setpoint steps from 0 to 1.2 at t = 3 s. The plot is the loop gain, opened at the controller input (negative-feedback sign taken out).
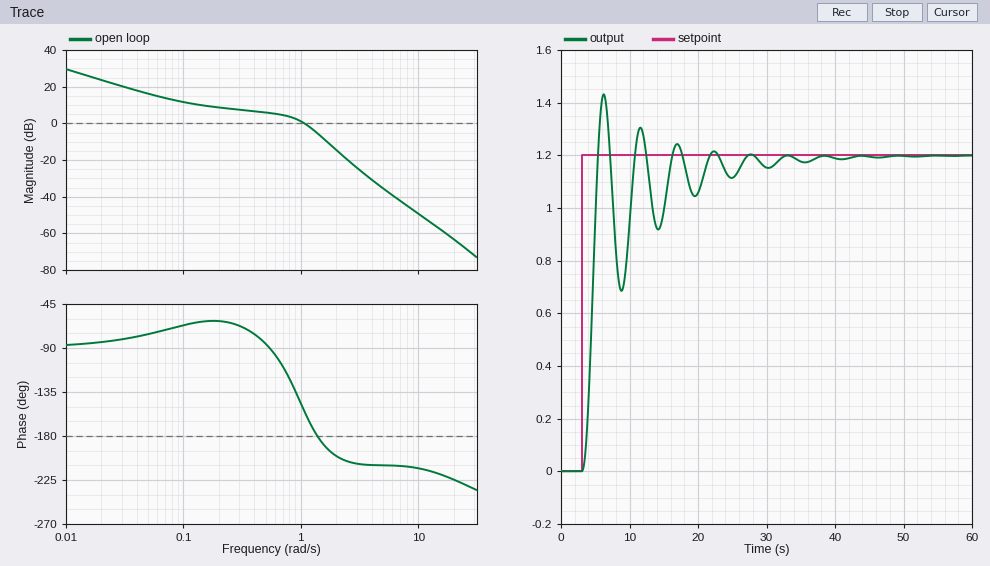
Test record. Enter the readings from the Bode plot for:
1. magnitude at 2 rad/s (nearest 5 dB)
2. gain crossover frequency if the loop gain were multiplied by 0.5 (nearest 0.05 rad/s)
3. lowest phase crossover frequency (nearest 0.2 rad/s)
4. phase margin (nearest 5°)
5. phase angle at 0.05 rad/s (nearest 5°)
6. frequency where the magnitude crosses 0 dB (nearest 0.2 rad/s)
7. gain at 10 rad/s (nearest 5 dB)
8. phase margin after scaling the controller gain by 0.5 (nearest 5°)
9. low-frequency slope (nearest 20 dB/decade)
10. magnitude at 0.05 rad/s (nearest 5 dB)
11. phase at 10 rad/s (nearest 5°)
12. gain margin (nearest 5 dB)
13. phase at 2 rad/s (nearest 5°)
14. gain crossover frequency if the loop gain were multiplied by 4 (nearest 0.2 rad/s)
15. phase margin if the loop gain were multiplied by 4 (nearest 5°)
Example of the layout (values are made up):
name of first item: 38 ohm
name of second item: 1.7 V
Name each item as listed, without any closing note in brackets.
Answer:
magnitude at 2 rad/s: -15 dB
gain crossover frequency if the loop gain were multiplied by 0.5: 0.50 rad/s
lowest phase crossover frequency: 1.4 rad/s
phase margin: 25°
phase angle at 0.05 rad/s: -75°
frequency where the magnitude crosses 0 dB: 1.0 rad/s
gain at 10 rad/s: -50 dB
phase margin after scaling the controller gain by 0.5: 95°
low-frequency slope: -20 dB/decade
magnitude at 0.05 rad/s: 15 dB
phase at 10 rad/s: -215°
gain margin: 5 dB
phase at 2 rad/s: -200°
gain crossover frequency if the loop gain were multiplied by 4: 1.8 rad/s
phase margin if the loop gain were multiplied by 4: -15°
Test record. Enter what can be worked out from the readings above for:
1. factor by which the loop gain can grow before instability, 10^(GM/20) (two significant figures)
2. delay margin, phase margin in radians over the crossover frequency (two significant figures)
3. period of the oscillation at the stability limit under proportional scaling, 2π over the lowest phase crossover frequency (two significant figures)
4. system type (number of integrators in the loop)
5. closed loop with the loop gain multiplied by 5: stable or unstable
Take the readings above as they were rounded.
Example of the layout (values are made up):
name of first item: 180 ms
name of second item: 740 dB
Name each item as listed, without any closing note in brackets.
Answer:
factor by which the loop gain can grow before instability, 10^(GM/20): 1.8
delay margin, phase margin in radians over the crossover frequency: 0.44 s
period of the oscillation at the stability limit under proportional scaling, 2π over the lowest phase crossover frequency: 4.5 s
system type: 1
closed loop with the loop gain multiplied by 5: stable or unstable: unstable
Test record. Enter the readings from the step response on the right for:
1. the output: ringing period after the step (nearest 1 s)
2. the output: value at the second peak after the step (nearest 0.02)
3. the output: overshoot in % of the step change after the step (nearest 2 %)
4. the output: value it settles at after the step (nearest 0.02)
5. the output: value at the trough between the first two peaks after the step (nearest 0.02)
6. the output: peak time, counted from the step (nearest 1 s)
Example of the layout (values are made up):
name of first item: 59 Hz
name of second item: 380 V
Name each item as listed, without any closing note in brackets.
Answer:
the output: ringing period after the step: 5 s
the output: value at the second peak after the step: 1.30
the output: overshoot in % of the step change after the step: 20 %
the output: value it settles at after the step: 1.20
the output: value at the trough between the first two peaks after the step: 0.68
the output: peak time, counted from the step: 3 s
